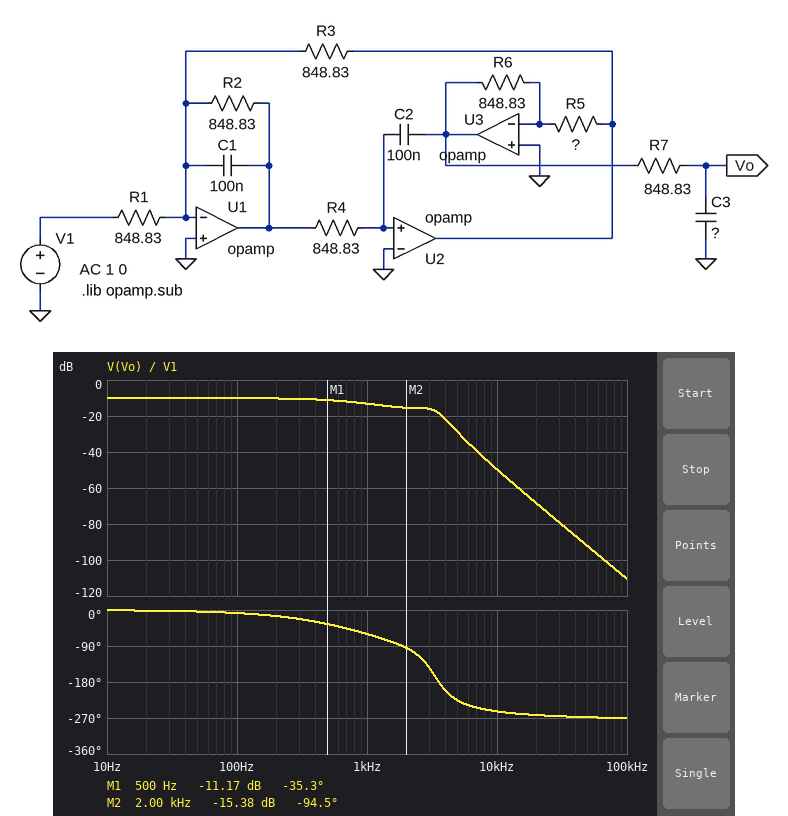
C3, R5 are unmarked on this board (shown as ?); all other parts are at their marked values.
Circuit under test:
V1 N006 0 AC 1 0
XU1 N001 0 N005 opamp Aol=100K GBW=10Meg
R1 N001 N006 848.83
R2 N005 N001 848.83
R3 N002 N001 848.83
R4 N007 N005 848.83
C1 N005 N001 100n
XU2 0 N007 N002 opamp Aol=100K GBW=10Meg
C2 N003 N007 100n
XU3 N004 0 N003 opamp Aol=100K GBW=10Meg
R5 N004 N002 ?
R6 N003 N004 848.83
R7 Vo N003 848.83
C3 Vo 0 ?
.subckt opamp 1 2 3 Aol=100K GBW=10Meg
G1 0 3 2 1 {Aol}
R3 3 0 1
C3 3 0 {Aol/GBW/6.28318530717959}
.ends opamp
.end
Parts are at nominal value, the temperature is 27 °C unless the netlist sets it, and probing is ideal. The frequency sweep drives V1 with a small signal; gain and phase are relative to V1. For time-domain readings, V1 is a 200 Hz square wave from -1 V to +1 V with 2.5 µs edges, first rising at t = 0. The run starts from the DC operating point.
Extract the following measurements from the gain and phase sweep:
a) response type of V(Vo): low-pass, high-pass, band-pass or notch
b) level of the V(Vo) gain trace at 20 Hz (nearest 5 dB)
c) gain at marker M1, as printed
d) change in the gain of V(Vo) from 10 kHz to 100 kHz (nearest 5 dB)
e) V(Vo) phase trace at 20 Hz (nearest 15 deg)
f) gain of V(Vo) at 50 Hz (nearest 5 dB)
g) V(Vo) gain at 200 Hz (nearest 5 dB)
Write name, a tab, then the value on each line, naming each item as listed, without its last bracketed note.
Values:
response type of V(Vo): low-pass, high-pass, band-pass or notch	low-pass
level of the V(Vo) gain trace at 20 Hz	-10 dB
gain at marker M1, as printed	-11.17 dB
change in the gain of V(Vo) from 10 kHz to 100 kHz	-60 dB
V(Vo) phase trace at 20 Hz	0 deg
gain of V(Vo) at 50 Hz	-10 dB
V(Vo) gain at 200 Hz	-10 dB
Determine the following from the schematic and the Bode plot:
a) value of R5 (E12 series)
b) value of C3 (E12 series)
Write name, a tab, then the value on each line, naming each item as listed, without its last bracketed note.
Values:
value of R5	2.7 kΩ
value of C3	220 nF
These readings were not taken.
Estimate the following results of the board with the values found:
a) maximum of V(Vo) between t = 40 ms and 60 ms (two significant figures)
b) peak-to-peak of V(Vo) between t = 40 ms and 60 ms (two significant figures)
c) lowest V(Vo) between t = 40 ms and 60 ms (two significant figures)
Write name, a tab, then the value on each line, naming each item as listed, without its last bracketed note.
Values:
maximum of V(Vo) between t = 40 ms and 60 ms	310 mV
peak-to-peak of V(Vo) between t = 40 ms and 60 ms	630 mV
lowest V(Vo) between t = 40 ms and 60 ms	-310 mV
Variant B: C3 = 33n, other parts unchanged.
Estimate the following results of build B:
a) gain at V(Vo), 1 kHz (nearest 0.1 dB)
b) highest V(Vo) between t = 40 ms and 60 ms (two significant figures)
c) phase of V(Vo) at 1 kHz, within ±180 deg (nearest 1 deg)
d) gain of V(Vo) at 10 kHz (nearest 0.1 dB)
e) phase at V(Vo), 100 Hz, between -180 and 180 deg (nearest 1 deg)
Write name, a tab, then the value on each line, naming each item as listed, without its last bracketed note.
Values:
gain at V(Vo), 1 kHz	-9.5 dB
highest V(Vo) between t = 40 ms and 60 ms	530 mV
phase of V(Vo) at 1 kHz, within ±180 deg	-20 deg
gain of V(Vo) at 10 kHz	-34.4 dB
phase at V(Vo), 100 Hz, between -180 and 180 deg	-2 deg
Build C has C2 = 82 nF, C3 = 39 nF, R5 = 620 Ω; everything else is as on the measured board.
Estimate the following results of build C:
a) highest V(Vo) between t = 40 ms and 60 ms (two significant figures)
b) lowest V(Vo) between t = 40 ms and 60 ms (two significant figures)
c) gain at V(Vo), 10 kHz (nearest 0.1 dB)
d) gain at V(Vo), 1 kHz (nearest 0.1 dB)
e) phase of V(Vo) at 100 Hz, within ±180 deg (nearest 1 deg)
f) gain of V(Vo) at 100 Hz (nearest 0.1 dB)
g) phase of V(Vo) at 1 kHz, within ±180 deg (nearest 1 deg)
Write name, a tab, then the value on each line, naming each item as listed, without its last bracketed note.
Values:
highest V(Vo) between t = 40 ms and 60 ms	1.7 V
lowest V(Vo) between t = 40 ms and 60 ms	-1.7 V
gain at V(Vo), 10 kHz	-34.5 dB
gain at V(Vo), 1 kHz	3.4 dB
phase of V(Vo) at 100 Hz, within ±180 deg	-5 deg
gain of V(Vo) at 100 Hz	2.7 dB
phase of V(Vo) at 1 kHz, within ±180 deg	-53 deg
